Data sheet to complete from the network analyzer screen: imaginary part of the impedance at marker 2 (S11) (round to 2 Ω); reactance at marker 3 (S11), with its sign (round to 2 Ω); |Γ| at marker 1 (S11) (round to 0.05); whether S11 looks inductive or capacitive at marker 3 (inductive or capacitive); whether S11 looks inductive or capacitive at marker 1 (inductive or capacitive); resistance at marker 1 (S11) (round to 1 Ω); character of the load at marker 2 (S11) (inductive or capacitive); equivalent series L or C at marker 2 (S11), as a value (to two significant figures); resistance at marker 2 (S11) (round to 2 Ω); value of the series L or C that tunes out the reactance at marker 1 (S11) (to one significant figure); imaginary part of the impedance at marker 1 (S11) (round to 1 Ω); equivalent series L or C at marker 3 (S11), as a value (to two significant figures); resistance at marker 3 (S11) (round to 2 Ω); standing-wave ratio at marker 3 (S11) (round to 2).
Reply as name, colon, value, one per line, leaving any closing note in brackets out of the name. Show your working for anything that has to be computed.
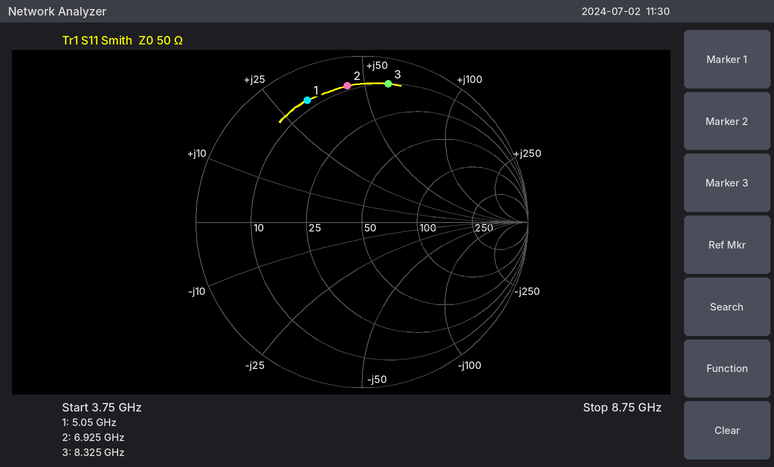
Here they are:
imaginary part of the impedance at marker 2 (S11): +44 Ω
reactance at marker 3 (S11), with its sign: +60 Ω
|Γ| at marker 1 (S11): 0.80
whether S11 looks inductive or capacitive at marker 3: inductive
whether S11 looks inductive or capacitive at marker 1: inductive
resistance at marker 1 (S11): 8 Ω
character of the load at marker 2 (S11): inductive
equivalent series L or C at marker 2 (S11), as a value: L = 44 Ω/(2π × 6.925 GHz) ≈ 1.0 nH
resistance at marker 2 (S11): 8 Ω
value of the series L or C that tunes out the reactance at marker 1 (S11): C = 1/(2π × 5.05 GHz × 32 Ω) ≈ 1.0 pF
imaginary part of the impedance at marker 1 (S11): +32 Ω
equivalent series L or C at marker 3 (S11), as a value: L = 60 Ω/(2π × 8.325 GHz) ≈ 1.1 nH
resistance at marker 3 (S11): 10 Ω
standing-wave ratio at marker 3 (S11): 12
